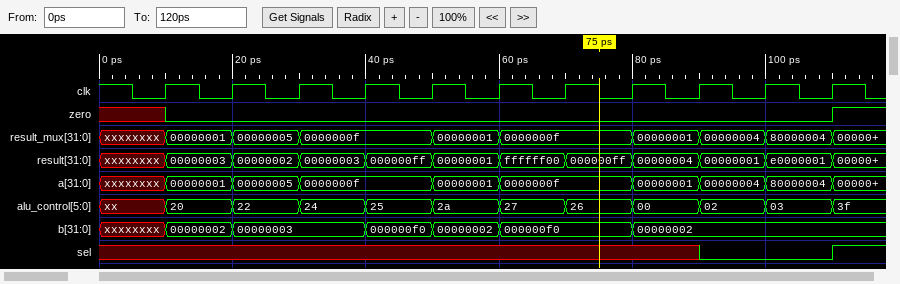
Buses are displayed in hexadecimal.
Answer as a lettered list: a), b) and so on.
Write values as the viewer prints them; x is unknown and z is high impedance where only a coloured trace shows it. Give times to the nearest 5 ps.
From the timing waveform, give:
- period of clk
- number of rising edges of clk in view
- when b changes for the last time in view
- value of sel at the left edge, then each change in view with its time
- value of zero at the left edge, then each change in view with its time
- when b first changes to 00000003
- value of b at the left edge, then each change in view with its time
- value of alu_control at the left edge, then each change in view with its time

a) 10 ps
b) 11
c) 80 ps
d) x, 0 at 90 ps, 1 at 110 ps
e) x, 0 at 10 ps, 1 at 110 ps
f) 20 ps
g) xxxxxxxx, 00000002 at 10 ps, 00000003 at 20 ps, 000000f0 at 40 ps, 00000002 at 50 ps, 000000f0 at 60 ps, 00000002 at 80 ps
h) xx, 20 at 10 ps, 22 at 20 ps, 24 at 30 ps, 25 at 40 ps, 2a at 50 ps, 27 at 60 ps, 26 at 70 ps, 00 at 80 ps, 02 at 90 ps, 03 at 100 ps, 3f at 110 ps
